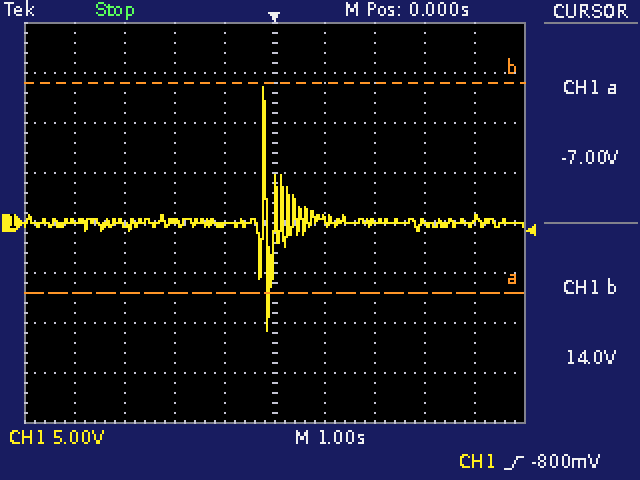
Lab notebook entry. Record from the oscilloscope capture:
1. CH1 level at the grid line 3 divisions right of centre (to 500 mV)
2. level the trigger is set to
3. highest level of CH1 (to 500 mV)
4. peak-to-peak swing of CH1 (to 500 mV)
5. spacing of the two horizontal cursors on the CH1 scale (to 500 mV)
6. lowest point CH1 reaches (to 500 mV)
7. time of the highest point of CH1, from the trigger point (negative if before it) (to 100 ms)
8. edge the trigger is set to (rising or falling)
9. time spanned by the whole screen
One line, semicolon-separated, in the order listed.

0.0 V; -800 mV; 13.5 V; 24.5 V; 21.0 V; -11.0 V; -200 ms; rising; 10 s
